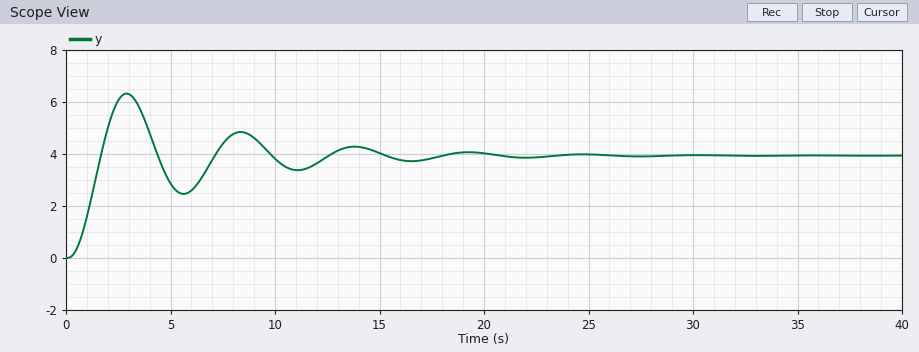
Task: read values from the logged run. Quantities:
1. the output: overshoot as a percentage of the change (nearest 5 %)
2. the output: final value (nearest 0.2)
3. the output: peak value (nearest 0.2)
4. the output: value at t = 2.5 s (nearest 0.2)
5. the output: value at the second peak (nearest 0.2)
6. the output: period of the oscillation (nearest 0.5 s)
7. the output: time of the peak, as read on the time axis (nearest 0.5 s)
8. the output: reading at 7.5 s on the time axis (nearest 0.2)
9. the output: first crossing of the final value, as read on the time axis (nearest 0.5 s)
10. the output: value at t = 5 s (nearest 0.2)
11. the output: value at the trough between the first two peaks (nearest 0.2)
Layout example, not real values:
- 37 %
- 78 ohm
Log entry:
- 60 %
- 4.0
- 6.4
- 6.0
- 4.8
- 5.5 s
- 3.0 s
- 4.4
- 1.5 s
- 2.8
- 2.4
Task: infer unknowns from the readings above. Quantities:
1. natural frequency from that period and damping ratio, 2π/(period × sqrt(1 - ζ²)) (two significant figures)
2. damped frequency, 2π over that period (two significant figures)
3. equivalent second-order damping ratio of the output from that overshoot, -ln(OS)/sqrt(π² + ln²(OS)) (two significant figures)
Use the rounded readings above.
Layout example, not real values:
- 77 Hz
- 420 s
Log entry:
- 1.2 rad/s
- 1.1 rad/s
- 0.16
